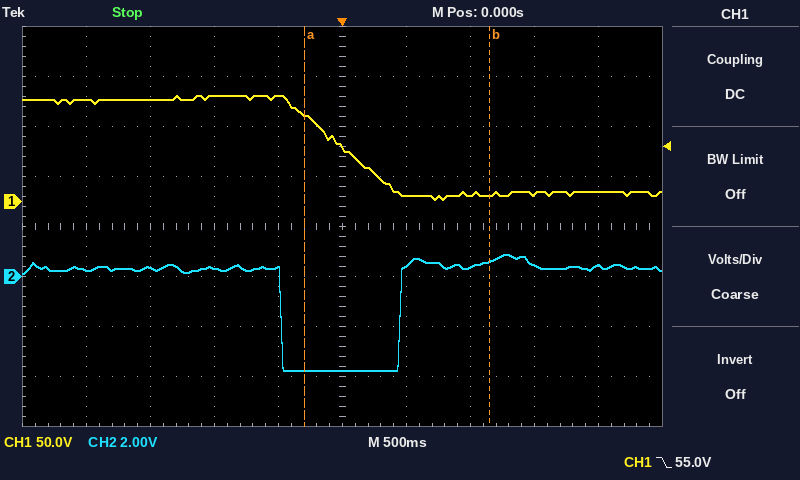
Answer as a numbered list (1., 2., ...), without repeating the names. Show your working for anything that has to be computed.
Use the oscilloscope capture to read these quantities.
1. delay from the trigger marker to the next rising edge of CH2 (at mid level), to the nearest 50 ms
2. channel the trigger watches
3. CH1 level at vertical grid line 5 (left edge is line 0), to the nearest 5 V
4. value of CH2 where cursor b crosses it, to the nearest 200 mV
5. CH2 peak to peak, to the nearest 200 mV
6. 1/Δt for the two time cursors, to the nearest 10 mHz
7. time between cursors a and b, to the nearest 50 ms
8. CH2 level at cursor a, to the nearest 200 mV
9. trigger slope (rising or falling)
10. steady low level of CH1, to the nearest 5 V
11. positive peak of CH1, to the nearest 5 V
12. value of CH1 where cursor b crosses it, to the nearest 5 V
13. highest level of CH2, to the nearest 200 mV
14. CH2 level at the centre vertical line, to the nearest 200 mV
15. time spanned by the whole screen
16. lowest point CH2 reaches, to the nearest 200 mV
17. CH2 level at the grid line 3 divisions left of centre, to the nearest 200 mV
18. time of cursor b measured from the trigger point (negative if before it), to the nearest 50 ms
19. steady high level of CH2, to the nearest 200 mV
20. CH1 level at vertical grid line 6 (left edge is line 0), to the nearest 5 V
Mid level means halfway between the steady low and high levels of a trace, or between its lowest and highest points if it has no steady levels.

1. 450 ms
2. CH1
3. 55 V
4. 600 mV
5. 800 mV − (-3.8 V) = 4.6 V
6. 1 / 1.45 s ≈ 690 mHz
7. 1.45 s
8. -3.8 V
9. falling
10. 10 V
11. 105 V
12. 5 V
13. 800 mV
14. -3.8 V
15. 5 s
16. -3.8 V
17. 400 mV
18. +1.15 s
19. 400 mV
20. 5 V
